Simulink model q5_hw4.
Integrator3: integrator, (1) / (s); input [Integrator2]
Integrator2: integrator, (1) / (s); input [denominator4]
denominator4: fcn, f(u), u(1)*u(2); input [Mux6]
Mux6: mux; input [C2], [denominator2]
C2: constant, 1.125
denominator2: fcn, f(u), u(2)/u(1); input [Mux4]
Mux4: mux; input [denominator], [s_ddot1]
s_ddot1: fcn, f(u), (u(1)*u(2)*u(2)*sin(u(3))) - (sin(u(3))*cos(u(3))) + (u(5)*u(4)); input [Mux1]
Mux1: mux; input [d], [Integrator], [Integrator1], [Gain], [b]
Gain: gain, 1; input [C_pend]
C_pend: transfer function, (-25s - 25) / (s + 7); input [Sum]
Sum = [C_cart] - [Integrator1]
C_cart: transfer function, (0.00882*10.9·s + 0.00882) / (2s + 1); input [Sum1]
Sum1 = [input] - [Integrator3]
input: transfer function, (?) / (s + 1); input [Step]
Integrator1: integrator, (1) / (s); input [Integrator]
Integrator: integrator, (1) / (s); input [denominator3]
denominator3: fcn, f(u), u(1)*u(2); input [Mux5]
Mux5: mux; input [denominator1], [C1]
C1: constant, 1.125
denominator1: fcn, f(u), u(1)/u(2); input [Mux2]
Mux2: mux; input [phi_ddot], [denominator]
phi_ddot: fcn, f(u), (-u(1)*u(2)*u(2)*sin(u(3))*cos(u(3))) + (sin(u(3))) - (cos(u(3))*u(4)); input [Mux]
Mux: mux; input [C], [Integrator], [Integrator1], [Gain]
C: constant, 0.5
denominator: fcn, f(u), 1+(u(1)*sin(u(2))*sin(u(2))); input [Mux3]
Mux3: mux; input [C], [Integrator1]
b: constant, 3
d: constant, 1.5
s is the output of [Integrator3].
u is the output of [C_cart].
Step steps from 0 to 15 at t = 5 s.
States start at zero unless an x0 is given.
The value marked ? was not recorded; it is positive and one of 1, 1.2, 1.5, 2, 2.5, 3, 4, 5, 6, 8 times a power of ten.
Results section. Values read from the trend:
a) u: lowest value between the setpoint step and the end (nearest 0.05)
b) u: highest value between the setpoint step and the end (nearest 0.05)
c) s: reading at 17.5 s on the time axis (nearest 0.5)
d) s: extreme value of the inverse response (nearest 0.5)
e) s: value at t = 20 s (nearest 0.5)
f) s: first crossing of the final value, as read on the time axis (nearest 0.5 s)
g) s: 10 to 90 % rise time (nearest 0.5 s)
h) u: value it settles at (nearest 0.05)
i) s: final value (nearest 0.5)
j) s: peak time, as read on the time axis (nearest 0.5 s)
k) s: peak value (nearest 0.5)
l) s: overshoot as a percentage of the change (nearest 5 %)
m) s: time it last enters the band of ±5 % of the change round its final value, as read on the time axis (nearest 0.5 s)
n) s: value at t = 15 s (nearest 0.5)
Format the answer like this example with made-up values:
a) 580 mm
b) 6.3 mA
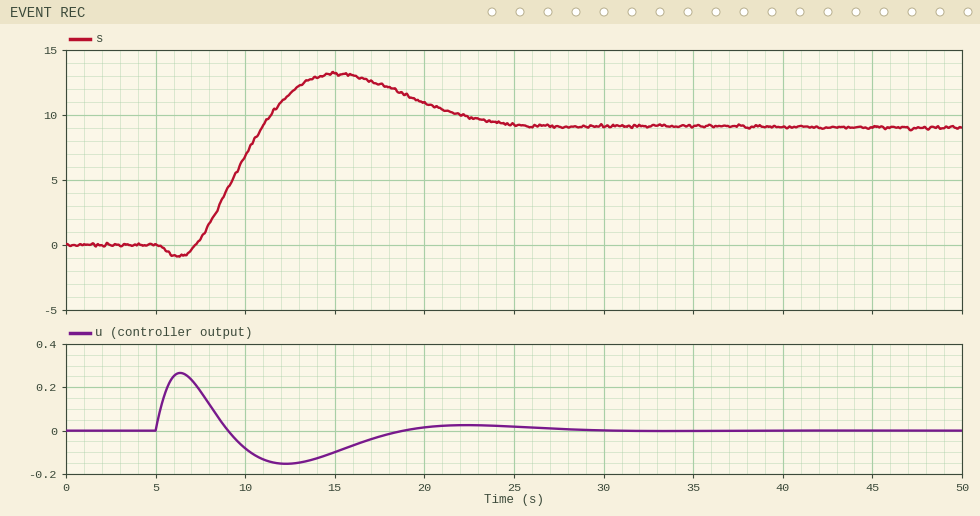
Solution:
a) -0.15
b) 0.25
c) 12.5
d) -1.0
e) 11.0
f) 11.0 s
g) 3.0 s
h) 0.00
i) 9.0
j) 15.0 s
k) 13.0
l) 45 %
m) 24.0 s
n) 13.0
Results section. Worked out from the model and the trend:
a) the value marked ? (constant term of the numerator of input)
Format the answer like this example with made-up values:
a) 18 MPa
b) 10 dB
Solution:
a) 0.6
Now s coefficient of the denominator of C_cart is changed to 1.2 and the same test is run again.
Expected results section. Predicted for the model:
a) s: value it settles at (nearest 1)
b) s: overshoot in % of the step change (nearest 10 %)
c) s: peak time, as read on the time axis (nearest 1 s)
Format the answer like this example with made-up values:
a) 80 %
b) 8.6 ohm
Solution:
a) 9
b) 40 %
c) 14 s
